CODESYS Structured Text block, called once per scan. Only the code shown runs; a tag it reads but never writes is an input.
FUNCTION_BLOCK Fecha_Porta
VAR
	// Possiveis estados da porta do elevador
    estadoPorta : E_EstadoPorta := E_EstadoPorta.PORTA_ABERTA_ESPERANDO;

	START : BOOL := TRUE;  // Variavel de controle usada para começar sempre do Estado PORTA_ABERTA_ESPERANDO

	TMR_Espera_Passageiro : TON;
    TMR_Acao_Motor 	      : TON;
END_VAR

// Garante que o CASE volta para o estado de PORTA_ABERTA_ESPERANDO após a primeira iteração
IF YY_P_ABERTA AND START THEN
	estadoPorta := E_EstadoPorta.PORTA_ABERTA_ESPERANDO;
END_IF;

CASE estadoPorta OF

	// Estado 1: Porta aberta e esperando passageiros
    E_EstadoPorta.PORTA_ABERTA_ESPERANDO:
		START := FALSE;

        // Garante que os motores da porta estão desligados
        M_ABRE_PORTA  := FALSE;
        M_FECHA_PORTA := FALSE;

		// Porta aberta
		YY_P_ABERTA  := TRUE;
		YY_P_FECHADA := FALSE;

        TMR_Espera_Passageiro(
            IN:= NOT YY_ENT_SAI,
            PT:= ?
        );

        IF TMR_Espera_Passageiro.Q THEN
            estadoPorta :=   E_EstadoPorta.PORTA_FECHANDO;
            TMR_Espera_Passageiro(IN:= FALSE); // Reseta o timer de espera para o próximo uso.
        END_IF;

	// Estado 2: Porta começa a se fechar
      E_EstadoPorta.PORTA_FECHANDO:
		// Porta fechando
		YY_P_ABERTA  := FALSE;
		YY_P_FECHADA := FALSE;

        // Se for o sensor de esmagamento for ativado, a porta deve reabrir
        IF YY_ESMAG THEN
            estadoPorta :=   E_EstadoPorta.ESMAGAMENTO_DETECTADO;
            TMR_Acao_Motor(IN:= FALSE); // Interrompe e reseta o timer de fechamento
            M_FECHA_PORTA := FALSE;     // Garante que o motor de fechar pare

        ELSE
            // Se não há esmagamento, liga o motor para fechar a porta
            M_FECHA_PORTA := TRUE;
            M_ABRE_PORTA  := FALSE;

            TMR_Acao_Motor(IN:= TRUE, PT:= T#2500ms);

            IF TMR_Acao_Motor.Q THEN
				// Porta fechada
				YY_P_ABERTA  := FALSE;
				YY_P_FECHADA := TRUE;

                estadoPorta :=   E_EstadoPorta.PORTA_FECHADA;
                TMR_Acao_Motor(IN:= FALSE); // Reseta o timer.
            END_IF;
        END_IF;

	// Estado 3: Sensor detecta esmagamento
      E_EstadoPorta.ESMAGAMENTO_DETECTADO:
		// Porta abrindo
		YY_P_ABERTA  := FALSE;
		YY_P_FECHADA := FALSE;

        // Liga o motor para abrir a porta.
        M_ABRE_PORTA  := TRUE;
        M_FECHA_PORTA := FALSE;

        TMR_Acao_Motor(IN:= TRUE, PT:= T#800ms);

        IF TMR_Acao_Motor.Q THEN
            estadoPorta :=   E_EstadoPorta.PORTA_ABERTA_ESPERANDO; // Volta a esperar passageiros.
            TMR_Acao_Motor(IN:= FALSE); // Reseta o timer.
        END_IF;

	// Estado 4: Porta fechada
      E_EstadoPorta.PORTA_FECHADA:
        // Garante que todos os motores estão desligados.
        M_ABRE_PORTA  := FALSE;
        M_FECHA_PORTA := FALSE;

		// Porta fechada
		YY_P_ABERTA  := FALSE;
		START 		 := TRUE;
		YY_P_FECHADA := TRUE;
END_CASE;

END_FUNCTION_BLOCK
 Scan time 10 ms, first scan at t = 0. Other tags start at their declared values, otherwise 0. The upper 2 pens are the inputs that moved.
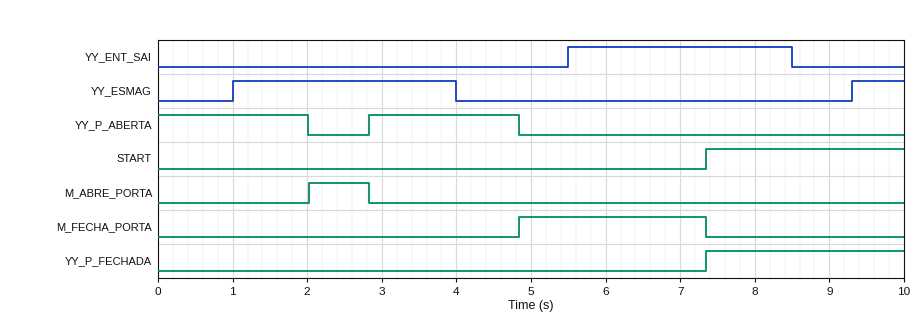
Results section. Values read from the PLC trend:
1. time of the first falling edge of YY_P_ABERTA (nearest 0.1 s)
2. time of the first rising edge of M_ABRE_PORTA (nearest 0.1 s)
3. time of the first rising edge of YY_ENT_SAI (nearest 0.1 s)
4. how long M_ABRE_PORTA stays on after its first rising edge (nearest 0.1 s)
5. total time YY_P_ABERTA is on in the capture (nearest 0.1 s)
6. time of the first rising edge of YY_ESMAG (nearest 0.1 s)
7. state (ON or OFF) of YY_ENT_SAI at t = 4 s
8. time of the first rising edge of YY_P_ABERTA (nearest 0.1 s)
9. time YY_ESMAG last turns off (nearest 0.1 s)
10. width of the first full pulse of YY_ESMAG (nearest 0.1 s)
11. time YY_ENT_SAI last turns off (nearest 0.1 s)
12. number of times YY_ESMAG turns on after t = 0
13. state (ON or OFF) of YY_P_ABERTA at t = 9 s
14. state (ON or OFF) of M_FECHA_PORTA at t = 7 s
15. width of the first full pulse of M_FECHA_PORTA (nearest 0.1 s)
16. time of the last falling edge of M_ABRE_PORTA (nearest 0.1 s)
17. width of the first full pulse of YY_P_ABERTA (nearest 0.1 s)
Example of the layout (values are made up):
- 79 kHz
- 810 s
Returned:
- 2.0 s
- 2.0 s
- 5.5 s
- 0.8 s
- 4.0 s
- 1.0 s
- OFF
- 2.8 s
- 4.0 s
- 3.0 s
- 8.5 s
- 2
- OFF
- ON
- 2.5 s
- 2.8 s
- 2.0 s
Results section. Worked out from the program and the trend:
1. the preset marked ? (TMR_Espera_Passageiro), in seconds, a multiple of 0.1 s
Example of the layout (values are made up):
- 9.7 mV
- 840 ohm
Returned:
- 2.0 s
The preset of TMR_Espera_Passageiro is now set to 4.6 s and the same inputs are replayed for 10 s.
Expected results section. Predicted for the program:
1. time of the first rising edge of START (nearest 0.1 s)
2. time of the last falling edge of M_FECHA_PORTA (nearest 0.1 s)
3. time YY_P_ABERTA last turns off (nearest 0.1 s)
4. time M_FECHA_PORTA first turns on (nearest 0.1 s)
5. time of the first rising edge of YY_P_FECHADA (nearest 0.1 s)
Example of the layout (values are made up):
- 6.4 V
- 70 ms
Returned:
- 7.1 s
- 7.1 s
- 4.6 s
- 4.6 s
- 7.1 s
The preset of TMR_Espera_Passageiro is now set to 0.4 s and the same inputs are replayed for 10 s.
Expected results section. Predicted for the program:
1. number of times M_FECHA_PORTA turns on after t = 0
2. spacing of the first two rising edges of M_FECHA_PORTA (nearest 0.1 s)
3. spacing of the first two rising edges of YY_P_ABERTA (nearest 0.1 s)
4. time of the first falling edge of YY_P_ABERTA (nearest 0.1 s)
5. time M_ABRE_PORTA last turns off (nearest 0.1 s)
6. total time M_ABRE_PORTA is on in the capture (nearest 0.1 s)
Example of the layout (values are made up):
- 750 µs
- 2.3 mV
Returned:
- 2
- 4.3 s
- 1.2 s
- 0.4 s
- 4.3 s
- 2.4 s
